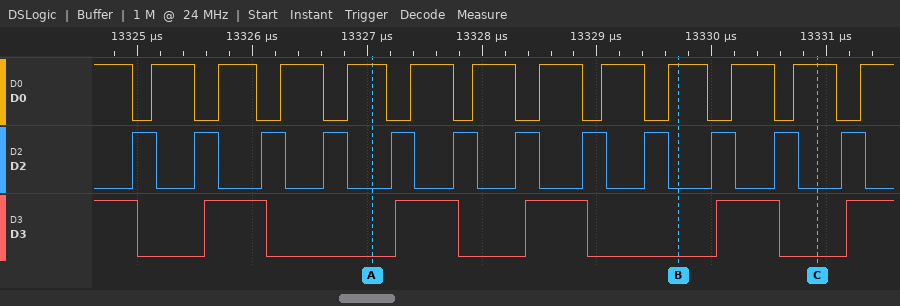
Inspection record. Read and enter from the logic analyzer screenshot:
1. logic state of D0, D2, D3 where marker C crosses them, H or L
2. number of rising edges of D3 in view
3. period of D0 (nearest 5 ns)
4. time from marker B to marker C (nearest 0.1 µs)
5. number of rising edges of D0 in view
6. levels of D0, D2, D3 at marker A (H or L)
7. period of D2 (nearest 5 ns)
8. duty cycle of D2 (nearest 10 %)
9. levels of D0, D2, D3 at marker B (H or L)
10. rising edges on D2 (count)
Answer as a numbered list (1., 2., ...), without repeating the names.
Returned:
1. D0=H, D2=L, D3=L
2. 5
3. 560 ns
4. 1.2 µs
5. 12
6. D0=H, D2=L, D3=L
7. 560 ns
8. 40 %
9. D0=H, D2=L, D3=L
10. 12
